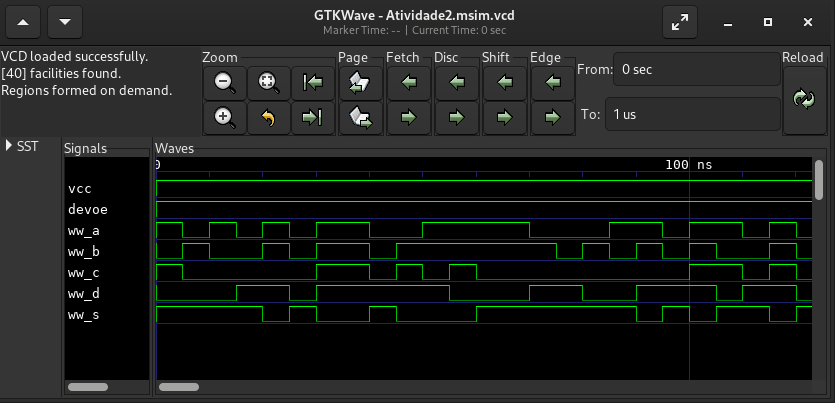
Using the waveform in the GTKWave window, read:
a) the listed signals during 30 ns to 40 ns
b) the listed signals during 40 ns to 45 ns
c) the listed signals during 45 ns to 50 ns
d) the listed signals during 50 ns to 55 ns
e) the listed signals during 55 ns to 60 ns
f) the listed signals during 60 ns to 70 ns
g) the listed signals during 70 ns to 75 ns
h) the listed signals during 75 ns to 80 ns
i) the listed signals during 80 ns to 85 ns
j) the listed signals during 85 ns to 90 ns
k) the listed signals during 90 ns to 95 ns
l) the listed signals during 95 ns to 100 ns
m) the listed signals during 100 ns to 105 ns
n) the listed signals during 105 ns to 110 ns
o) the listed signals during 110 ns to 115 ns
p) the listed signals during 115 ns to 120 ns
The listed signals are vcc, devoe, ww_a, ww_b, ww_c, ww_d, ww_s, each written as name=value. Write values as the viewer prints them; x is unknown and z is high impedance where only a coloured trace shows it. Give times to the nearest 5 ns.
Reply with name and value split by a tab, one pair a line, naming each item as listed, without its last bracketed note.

the listed signals during 30 ns to 40 ns	vcc=1, devoe=1, ww_a=1, ww_b=1, ww_c=1, ww_d=1, ww_s=0
the listed signals during 40 ns to 45 ns	vcc=1, devoe=1, ww_a=0, ww_b=0, ww_c=0, ww_d=1, ww_s=1
the listed signals during 45 ns to 50 ns	vcc=1, devoe=1, ww_a=0, ww_b=1, ww_c=1, ww_d=1, ww_s=0
the listed signals during 50 ns to 55 ns	vcc=1, devoe=1, ww_a=1, ww_b=1, ww_c=0, ww_d=1, ww_s=0
the listed signals during 55 ns to 60 ns	vcc=1, devoe=1, ww_a=1, ww_b=1, ww_c=1, ww_d=0, ww_s=0
the listed signals during 60 ns to 70 ns	vcc=1, devoe=1, ww_a=1, ww_b=1, ww_c=0, ww_d=0, ww_s=1
the listed signals during 70 ns to 75 ns	vcc=1, devoe=1, ww_a=0, ww_b=1, ww_c=0, ww_d=1, ww_s=1
the listed signals during 75 ns to 80 ns	vcc=1, devoe=1, ww_a=0, ww_b=0, ww_c=0, ww_d=1, ww_s=1
the listed signals during 80 ns to 85 ns	vcc=1, devoe=1, ww_a=0, ww_b=1, ww_c=0, ww_d=0, ww_s=1
the listed signals during 85 ns to 90 ns	vcc=1, devoe=1, ww_a=1, ww_b=0, ww_c=0, ww_d=0, ww_s=1
the listed signals during 90 ns to 95 ns	vcc=1, devoe=1, ww_a=1, ww_b=1, ww_c=0, ww_d=1, ww_s=0
the listed signals during 95 ns to 100 ns	vcc=1, devoe=1, ww_a=0, ww_b=0, ww_c=0, ww_d=1, ww_s=1
the listed signals during 100 ns to 105 ns	vcc=1, devoe=1, ww_a=1, ww_b=1, ww_c=1, ww_d=1, ww_s=0
the listed signals during 105 ns to 110 ns	vcc=1, devoe=1, ww_a=1, ww_b=0, ww_c=1, ww_d=0, ww_s=1
the listed signals during 110 ns to 115 ns	vcc=1, devoe=1, ww_a=0, ww_b=0, ww_c=0, ww_d=1, ww_s=1
the listed signals during 115 ns to 120 ns	vcc=1, devoe=1, ww_a=1, ww_b=1, ww_c=1, ww_d=1, ww_s=0
